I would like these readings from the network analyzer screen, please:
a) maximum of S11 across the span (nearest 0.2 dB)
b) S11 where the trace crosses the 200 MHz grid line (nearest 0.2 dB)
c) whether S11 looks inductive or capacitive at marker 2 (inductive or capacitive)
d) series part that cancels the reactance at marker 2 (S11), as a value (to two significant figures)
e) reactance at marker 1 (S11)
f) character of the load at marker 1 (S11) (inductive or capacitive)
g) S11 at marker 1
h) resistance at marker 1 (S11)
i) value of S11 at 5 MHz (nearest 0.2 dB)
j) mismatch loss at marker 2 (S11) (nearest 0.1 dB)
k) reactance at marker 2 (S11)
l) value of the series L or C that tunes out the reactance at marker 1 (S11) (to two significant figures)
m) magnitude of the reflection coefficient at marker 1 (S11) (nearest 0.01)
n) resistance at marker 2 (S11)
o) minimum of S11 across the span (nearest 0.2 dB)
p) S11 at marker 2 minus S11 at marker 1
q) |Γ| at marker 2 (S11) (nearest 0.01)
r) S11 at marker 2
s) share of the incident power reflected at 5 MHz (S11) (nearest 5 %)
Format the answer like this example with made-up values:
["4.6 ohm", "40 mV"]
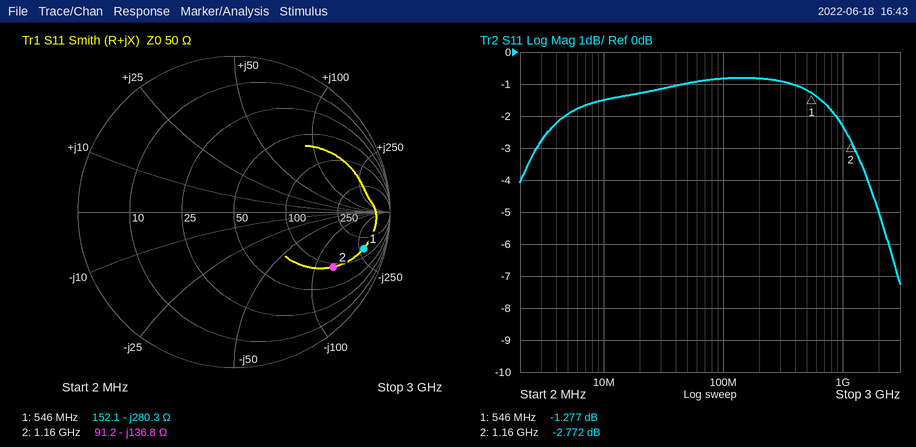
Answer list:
["-0.8 dB", "-0.8 dB", "capacitive", "19 nH", "-280.3 Ω", "capacitive", "-1.277 dB", "152.1 Ω", "-2.0 dB", "3.3 dB", "-136.8 Ω", "82 nH", "0.86", "91.2 Ω", "-7.2 dB", "-1.495 dB", "0.73", "-2.772 dB", "65 %"]
